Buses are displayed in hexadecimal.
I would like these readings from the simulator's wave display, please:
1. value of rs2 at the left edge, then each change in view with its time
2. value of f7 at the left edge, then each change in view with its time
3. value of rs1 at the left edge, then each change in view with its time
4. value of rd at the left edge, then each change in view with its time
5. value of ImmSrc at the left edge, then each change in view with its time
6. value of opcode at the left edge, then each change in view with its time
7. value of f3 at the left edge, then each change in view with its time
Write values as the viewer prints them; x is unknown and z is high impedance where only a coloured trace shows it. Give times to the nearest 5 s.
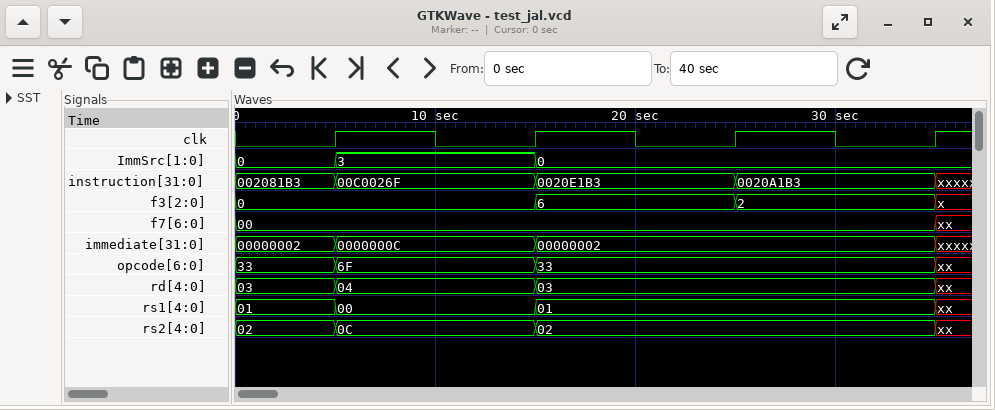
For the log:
02, 0C at 5 s, 02 at 15 s, xx at 35 s
00, xx at 35 s
01, 00 at 5 s, 01 at 15 s, xx at 35 s
03, 04 at 5 s, 03 at 15 s, xx at 35 s
0, 3 at 5 s, 0 at 15 s
33, 6F at 5 s, 33 at 15 s, xx at 35 s
0, 6 at 15 s, 2 at 25 s, x at 35 s
